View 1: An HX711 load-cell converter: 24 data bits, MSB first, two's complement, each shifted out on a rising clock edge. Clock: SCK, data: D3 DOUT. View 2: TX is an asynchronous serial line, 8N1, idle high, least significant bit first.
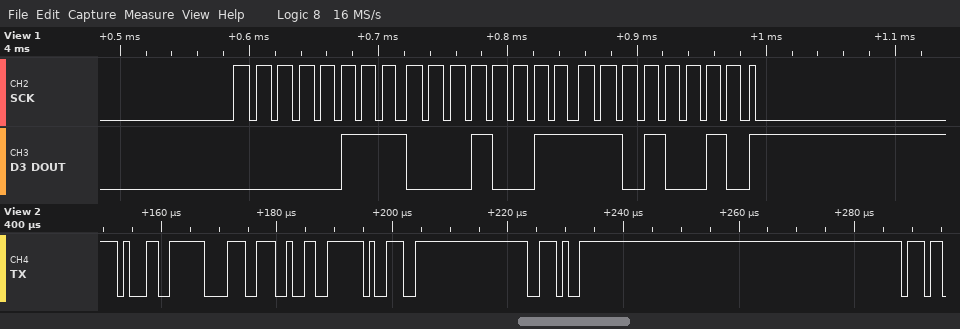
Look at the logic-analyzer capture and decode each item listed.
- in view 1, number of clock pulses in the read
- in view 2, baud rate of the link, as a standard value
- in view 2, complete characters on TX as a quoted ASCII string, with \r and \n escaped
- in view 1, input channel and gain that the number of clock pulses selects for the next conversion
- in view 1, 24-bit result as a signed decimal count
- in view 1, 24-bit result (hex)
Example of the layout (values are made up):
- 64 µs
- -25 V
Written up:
- 25
- 1000000 baud
- "1829."
- channel A, gain 128
- 463826
- 0x0713D2
